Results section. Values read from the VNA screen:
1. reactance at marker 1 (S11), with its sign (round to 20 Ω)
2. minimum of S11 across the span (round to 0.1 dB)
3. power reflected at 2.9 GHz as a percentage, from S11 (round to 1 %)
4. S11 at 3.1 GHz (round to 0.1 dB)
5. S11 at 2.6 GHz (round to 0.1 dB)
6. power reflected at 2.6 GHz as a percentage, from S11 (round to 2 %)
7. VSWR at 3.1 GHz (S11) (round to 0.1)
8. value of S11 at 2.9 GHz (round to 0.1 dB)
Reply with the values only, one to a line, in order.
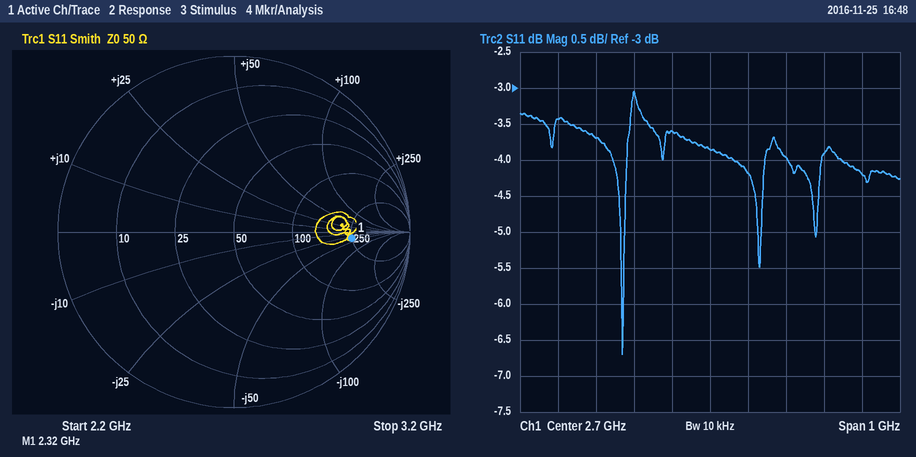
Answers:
-40 Ω
-6.7 dB
40 %
-4.2 dB
-3.6 dB
44 %
4.2
-4.0 dB
